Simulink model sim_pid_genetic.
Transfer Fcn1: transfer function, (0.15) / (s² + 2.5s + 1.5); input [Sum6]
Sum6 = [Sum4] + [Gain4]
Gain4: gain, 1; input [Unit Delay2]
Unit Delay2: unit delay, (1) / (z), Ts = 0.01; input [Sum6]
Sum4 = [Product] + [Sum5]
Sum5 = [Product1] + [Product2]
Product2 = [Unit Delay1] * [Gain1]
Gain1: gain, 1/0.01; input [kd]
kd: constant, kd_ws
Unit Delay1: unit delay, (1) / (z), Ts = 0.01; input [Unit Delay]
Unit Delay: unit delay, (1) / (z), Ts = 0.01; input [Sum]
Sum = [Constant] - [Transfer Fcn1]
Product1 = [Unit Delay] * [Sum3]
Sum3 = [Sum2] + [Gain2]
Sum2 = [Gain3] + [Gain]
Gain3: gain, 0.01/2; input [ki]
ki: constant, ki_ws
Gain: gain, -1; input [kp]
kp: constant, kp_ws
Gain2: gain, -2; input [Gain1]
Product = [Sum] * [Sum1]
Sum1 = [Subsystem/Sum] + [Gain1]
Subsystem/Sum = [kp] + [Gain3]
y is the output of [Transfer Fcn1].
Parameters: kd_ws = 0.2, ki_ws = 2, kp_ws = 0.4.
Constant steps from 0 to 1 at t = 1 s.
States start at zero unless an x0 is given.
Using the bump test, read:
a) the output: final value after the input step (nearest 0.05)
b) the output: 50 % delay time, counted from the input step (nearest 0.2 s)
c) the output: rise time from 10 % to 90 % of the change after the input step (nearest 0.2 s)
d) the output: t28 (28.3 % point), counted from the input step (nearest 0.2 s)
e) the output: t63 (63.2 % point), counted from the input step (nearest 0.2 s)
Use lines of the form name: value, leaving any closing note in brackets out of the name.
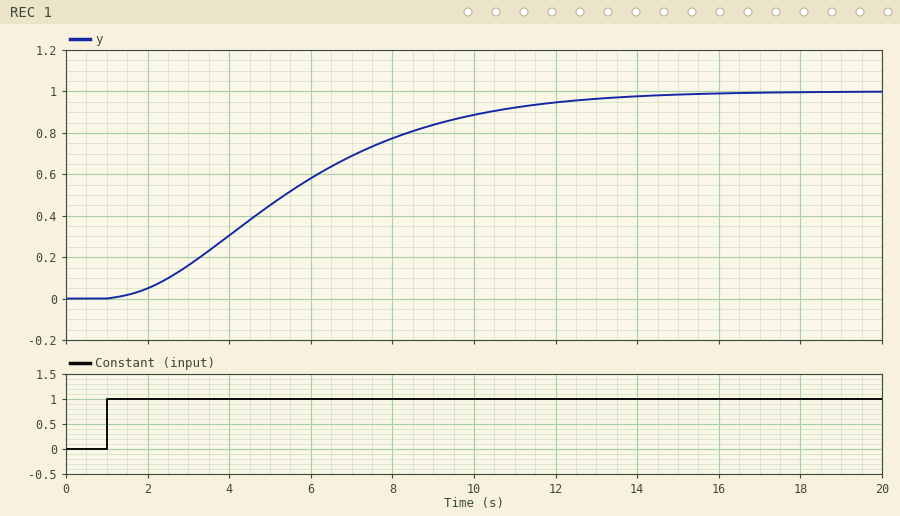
the output: final value after the input step: 1.00
the output: 50 % delay time, counted from the input step: 4.4 s
the output: rise time from 10 % to 90 % of the change after the input step: 7.8 s
the output: t28 (28.3 % point), counted from the input step: 2.8 s
the output: t63 (63.2 % point), counted from the input step: 5.4 s
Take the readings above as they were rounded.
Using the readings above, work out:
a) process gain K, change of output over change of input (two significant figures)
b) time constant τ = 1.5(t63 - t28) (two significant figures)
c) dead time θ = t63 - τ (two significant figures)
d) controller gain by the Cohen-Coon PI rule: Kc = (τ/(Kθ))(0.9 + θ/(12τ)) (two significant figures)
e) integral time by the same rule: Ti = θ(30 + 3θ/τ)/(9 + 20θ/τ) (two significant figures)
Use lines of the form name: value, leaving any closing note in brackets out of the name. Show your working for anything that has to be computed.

process gain K, change of output over change of input: (1 - 0) / 1 = 1.0
time constant τ = 1.5(t63 - t28): 1.5 × (5.4 - 2.8) = 3.9 s
dead time θ = t63 - τ: 5.4 - 3.9 = 1.5 s
controller gain by the Cohen-Coon PI rule: Kc = (τ/(Kθ))(0.9 + θ/(12τ)): 3.9 / (1 × 1.5) × (0.9 + 1.5 / (12 × 3.9)) = 2.4
integral time by the same rule: Ti = θ(30 + 3θ/τ)/(9 + 20θ/τ): 1.5 × (30 + 3 × 1.5 / 3.9) / (9 + 20 × 1.5 / 3.9) = 2.8 s
